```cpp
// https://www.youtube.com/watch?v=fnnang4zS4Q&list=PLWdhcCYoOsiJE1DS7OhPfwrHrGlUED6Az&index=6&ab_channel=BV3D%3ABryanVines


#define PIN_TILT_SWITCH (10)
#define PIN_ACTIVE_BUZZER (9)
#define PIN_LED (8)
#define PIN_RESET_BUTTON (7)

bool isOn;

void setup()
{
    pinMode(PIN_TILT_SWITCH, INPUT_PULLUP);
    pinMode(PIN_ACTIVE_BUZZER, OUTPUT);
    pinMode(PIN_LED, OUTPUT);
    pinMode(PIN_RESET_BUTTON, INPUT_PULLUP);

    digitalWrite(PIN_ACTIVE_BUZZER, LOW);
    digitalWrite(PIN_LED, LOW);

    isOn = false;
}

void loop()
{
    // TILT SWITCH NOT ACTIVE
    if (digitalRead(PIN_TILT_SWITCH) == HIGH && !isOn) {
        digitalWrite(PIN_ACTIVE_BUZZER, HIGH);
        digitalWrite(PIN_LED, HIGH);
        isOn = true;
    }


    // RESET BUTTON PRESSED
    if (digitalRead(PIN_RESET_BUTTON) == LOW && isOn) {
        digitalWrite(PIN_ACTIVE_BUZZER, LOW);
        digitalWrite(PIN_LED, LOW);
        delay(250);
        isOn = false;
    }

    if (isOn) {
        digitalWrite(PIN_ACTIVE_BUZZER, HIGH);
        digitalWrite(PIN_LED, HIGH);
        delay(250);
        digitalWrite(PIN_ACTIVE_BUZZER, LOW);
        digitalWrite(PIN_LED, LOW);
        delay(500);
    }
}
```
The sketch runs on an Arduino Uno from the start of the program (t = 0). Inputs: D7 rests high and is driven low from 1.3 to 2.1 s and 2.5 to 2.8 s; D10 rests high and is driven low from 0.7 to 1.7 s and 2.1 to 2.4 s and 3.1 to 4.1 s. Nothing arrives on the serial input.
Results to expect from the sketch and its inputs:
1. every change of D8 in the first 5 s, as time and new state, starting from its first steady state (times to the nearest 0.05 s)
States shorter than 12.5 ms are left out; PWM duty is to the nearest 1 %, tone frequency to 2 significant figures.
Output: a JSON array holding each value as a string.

["0 s high; 0.25 s low; 0.75 s high; 1 s low; 2.4 s high; 2.65 s low; 3.15 s high; 3.4 s low; 3.9 s high; 4.15 s low; 4.65 s high; 4.9 s low"]
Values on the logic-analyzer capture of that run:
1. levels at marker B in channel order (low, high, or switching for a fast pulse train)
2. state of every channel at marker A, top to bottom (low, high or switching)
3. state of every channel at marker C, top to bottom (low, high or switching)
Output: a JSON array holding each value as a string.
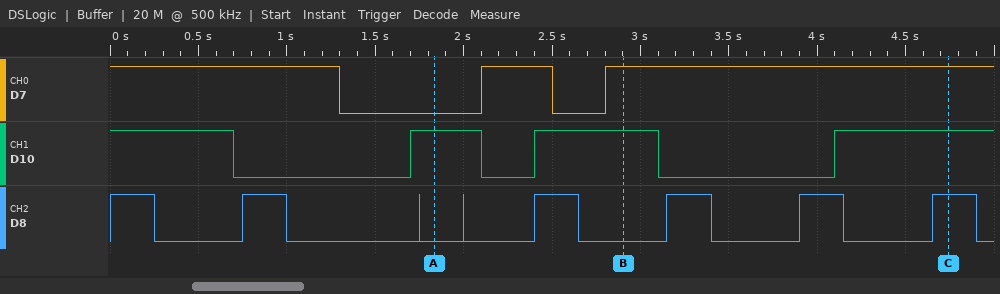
["D7 high, D10 high, D8 low", "D7 low, D10 high, D8 low", "D7 high, D10 high, D8 high"]
